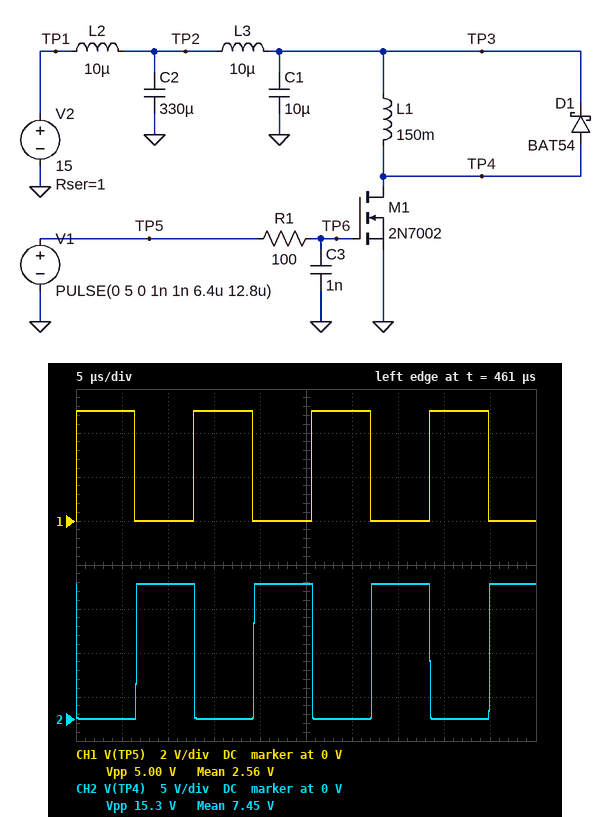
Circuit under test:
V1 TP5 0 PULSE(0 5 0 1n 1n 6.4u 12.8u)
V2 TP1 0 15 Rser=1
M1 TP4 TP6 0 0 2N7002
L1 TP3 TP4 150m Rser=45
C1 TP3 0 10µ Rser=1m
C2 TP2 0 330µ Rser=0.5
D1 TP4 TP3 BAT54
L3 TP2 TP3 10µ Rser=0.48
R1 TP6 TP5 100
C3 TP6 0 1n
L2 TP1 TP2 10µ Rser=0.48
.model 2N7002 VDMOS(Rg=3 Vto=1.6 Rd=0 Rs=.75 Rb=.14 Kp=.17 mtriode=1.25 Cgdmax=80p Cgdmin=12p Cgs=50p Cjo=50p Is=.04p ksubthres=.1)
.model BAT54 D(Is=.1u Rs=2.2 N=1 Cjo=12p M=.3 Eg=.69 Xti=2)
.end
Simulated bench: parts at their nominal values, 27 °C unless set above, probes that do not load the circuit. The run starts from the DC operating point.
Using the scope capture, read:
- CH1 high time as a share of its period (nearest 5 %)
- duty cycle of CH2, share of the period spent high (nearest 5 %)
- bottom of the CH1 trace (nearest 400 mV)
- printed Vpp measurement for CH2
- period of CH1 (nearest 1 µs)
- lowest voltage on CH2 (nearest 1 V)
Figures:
50 %
50 %
0 V
15.3 V
13 µs
0 V
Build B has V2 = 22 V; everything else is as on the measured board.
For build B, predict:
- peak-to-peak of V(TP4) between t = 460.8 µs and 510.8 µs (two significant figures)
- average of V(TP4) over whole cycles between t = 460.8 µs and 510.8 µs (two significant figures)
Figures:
22 V
11 V
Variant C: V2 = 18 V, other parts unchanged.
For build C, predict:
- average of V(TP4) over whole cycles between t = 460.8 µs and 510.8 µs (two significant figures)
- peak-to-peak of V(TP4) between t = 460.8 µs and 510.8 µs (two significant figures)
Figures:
9.1 V
18 V
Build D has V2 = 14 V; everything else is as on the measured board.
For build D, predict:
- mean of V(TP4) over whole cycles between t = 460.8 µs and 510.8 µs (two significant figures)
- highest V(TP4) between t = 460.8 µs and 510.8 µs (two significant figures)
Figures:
7.1 V
14 V
